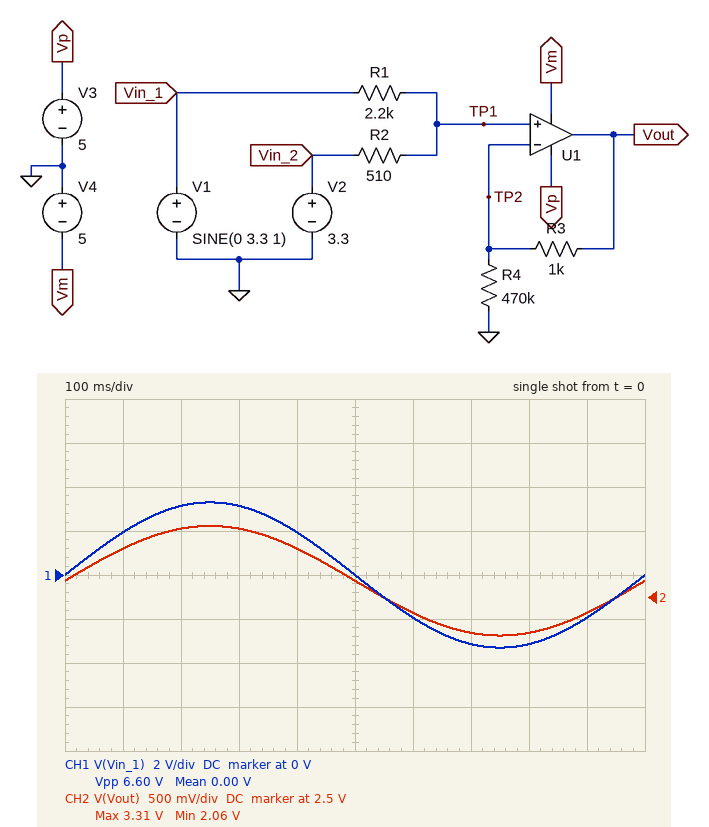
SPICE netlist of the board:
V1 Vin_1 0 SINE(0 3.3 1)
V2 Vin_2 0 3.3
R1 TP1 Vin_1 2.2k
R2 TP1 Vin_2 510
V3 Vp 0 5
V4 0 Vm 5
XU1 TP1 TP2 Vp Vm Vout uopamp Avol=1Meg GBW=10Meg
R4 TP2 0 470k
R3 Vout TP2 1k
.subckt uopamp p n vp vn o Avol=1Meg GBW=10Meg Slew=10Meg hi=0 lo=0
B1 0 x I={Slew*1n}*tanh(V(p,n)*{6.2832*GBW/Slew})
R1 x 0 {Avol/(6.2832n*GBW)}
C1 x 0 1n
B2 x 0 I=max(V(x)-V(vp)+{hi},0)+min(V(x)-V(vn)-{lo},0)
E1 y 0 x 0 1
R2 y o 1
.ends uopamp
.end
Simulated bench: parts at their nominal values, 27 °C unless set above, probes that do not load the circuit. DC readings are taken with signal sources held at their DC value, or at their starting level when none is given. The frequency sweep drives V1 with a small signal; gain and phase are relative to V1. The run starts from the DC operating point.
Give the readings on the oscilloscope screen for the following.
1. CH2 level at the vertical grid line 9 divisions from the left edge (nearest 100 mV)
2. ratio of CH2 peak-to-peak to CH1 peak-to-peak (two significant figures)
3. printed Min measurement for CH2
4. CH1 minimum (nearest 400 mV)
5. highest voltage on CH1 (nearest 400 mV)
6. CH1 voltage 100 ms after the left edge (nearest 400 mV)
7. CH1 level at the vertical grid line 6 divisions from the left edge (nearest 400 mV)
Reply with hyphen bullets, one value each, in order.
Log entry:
- 2.3 V
- 0.19
- 2.06 V
- -3.2 V
- 3.2 V
- 2.0 V
- -2.0 V
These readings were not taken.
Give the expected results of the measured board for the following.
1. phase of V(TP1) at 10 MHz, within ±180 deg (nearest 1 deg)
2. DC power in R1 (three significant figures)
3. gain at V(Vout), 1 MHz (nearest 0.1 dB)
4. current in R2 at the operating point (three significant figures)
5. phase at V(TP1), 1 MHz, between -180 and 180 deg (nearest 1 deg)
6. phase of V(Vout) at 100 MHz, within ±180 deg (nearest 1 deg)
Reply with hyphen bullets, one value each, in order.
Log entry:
- 0 deg
- 3.26 mW
- -14.5 dB
- 1.22 mA
- 0 deg
- -84 deg
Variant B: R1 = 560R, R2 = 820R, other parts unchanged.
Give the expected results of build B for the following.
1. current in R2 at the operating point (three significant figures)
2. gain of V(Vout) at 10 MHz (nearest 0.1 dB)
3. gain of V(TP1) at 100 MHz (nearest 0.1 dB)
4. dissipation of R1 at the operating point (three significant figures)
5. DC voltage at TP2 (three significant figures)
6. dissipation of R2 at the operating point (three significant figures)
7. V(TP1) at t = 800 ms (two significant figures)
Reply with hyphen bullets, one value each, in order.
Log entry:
- 2.39 mA
- -7.5 dB
- -4.5 dB
- 3.20 mW
- 1.34 V
- 4.69 mW
- -530 mV
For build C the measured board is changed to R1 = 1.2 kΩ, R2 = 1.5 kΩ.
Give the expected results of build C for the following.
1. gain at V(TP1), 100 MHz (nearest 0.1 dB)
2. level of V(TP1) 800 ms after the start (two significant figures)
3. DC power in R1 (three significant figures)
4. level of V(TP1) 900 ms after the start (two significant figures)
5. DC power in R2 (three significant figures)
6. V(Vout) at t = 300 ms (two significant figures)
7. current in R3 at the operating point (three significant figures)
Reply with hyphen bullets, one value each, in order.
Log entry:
- -5.1 dB
- -280 mV
- 1.79 mW
- 390 mV
- 2.24 mW
- 3.2 V
- 3.12 µA
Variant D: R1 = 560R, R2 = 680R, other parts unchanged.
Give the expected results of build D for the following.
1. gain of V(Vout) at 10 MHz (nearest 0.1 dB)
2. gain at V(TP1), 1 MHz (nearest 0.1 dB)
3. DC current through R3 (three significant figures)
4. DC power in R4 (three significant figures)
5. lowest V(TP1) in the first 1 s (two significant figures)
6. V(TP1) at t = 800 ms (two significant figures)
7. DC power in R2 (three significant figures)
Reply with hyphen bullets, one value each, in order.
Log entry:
- -8.2 dB
- -5.2 dB
- 3.17 µA
- 4.73 µW
- -320 mV
- -230 mV
- 4.82 mW
